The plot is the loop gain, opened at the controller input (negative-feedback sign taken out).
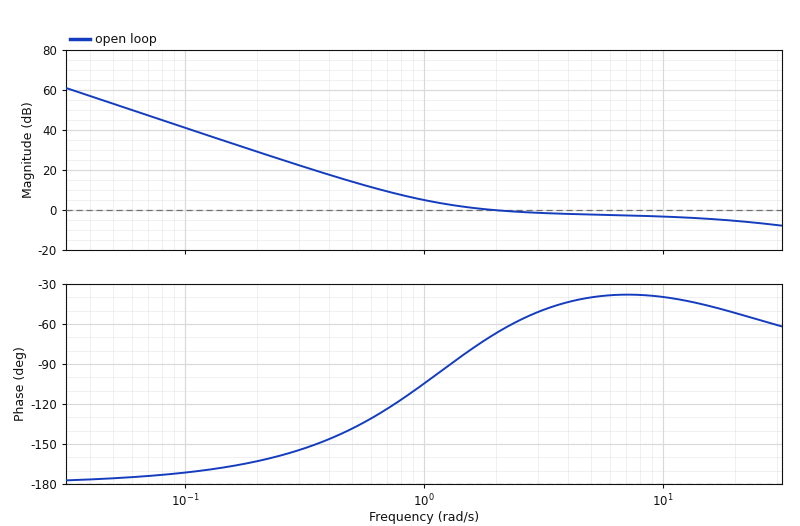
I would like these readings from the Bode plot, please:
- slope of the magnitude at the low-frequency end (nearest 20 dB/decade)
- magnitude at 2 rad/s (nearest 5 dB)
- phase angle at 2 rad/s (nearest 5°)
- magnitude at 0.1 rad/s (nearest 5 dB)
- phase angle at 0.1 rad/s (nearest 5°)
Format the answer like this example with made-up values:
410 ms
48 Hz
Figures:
-40 dB/decade
0 dB
-65°
40 dB
-170°
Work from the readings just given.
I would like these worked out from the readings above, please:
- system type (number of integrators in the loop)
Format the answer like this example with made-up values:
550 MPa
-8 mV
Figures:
2
